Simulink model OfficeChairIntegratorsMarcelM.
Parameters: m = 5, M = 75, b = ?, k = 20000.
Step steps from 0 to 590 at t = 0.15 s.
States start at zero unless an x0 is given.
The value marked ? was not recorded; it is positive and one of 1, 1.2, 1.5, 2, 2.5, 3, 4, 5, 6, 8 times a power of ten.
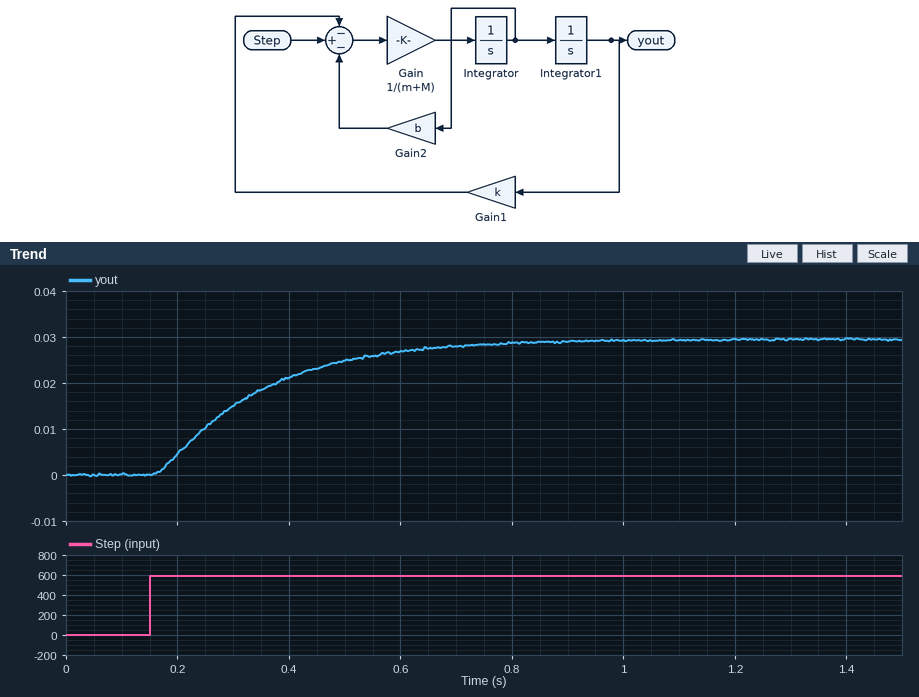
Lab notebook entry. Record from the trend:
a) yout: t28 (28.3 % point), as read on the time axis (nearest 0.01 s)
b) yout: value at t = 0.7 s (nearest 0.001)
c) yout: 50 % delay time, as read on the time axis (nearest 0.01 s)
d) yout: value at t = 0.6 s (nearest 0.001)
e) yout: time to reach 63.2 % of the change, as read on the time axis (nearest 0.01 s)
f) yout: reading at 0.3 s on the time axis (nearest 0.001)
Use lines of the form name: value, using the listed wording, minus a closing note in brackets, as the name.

yout: t28 (28.3 % point), as read on the time axis: 0.23 s
yout: value at t = 0.7 s: 0.028
yout: 50 % delay time, as read on the time axis: 0.30 s
yout: value at t = 0.6 s: 0.027
yout: time to reach 63.2 % of the change, as read on the time axis: 0.35 s
yout: reading at 0.3 s on the time axis: 0.015
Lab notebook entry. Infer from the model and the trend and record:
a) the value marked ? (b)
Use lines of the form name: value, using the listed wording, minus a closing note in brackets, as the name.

the value marked ?: 4000
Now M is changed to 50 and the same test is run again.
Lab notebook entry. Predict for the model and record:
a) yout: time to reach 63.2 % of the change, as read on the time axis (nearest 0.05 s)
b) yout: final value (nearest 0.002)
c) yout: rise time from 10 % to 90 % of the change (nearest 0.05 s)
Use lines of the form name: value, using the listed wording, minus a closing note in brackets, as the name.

yout: time to reach 63.2 % of the change, as read on the time axis: 0.35 s
yout: final value: 0.030
yout: rise time from 10 % to 90 % of the change: 0.40 s
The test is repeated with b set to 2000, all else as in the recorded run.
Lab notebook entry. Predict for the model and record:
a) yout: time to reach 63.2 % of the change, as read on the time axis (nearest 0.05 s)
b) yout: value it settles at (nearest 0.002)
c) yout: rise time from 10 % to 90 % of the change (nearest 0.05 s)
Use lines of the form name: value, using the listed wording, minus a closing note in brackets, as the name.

yout: time to reach 63.2 % of the change, as read on the time axis: 0.25 s
yout: value it settles at: 0.030
yout: rise time from 10 % to 90 % of the change: 0.15 s
